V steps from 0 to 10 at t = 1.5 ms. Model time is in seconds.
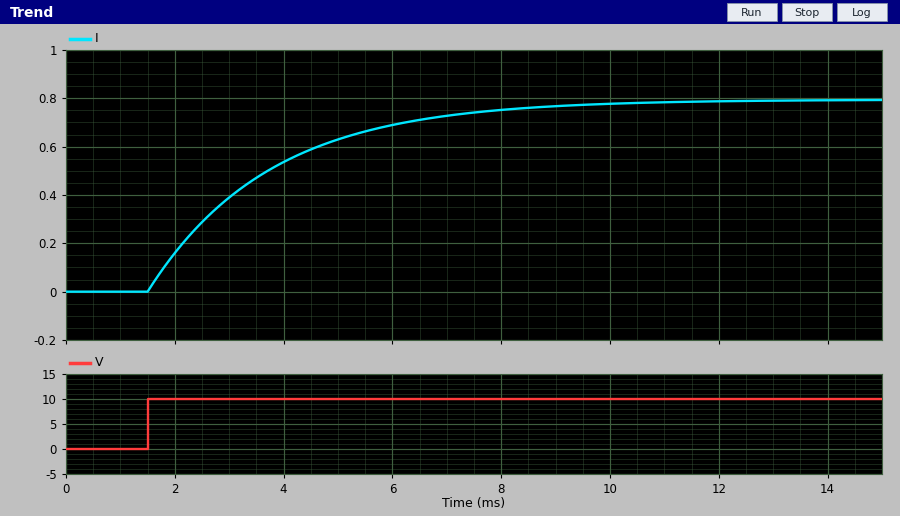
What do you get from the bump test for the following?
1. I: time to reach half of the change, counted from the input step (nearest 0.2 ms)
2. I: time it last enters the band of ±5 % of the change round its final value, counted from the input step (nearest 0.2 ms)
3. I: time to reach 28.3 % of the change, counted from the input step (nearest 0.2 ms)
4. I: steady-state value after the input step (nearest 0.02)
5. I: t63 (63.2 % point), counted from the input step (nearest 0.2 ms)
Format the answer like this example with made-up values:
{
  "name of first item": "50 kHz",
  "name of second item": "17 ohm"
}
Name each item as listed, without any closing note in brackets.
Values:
{
  "I: time to reach half of the change, counted from the input step": "1.6 ms",
  "I: time it last enters the band of ±5 % of the change round its final value, counted from the input step": "6.6 ms",
  "I: time to reach 28.3 % of the change, counted from the input step": "0.8 ms",
  "I: steady-state value after the input step": "0.80",
  "I: t63 (63.2 % point), counted from the input step": "2.2 ms"
}
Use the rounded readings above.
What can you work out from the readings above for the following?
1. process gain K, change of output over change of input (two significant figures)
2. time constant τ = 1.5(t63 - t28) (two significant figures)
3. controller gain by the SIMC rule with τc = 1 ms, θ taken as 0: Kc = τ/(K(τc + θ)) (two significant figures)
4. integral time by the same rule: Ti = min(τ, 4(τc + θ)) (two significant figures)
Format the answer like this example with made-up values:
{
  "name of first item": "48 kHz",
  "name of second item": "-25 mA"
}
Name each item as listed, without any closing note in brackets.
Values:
{
  "process gain K, change of output over change of input": "0.080",
  "time constant τ = 1.5(t63 - t28)": "2.1 ms",
  "controller gain by the SIMC rule with τc = 1 ms, θ taken as 0: Kc = τ/(K(τc + θ))": "26",
  "integral time by the same rule: Ti = min(τ, 4(τc + θ))": "2.1 ms"
}
